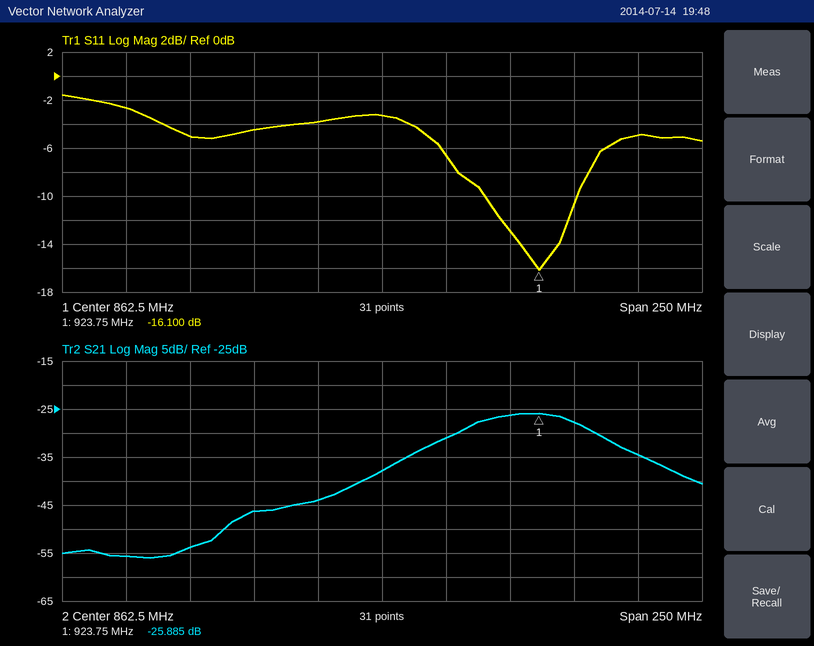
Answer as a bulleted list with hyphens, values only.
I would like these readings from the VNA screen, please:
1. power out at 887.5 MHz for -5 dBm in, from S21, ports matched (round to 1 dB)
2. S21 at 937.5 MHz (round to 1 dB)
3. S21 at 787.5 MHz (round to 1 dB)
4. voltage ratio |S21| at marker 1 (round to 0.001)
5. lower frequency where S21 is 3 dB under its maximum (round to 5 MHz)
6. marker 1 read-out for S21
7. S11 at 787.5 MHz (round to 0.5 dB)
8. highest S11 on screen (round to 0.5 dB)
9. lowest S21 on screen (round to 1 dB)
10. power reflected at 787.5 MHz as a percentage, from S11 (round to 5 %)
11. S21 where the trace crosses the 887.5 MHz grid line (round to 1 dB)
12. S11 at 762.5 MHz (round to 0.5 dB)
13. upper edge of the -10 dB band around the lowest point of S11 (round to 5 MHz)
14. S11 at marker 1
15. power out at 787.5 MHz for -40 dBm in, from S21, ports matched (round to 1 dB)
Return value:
- -36 dBm
- -28 dB
- -54 dB
- 0.051
- 895 MHz
- -25.885 dB
- -5.0 dB
- -1.5 dB
- -56 dB
- 30 %
- -31 dB
- -2.5 dB
- 940 MHz
- -16.100 dB
- -94 dBm
